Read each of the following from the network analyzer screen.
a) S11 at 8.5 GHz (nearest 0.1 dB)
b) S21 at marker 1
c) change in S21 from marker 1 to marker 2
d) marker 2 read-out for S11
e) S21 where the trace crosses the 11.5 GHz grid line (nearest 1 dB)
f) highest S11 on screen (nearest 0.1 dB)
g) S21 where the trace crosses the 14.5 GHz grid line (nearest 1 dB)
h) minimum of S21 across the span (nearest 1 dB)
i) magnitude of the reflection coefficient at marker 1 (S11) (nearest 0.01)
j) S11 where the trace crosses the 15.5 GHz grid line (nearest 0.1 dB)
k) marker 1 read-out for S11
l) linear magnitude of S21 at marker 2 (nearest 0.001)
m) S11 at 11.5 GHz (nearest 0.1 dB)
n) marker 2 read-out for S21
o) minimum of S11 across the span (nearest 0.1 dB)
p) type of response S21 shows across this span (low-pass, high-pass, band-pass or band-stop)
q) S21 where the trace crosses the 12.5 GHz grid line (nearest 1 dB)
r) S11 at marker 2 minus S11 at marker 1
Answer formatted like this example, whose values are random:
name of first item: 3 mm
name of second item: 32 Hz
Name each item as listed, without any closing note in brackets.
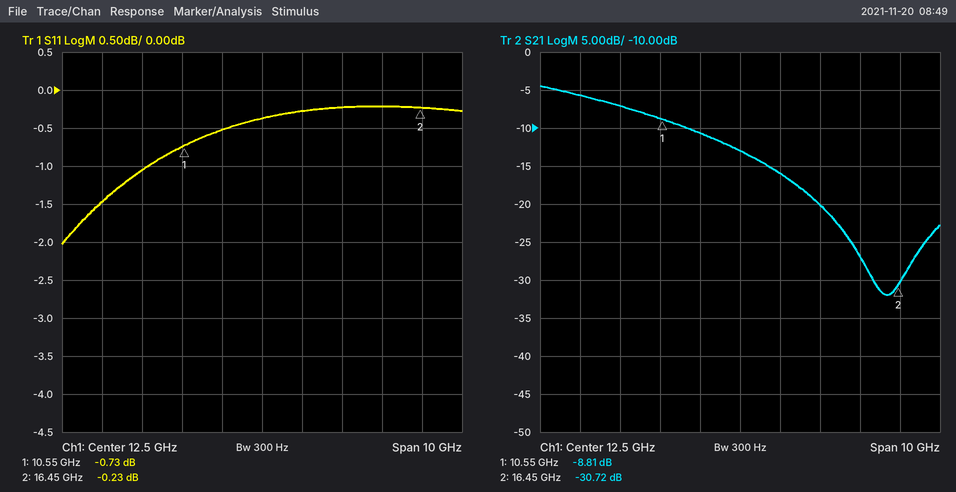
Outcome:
S11 at 8.5 GHz: -1.5 dB
S21 at marker 1: -8.81 dB
change in S21 from marker 1 to marker 2: -21.91 dB
marker 2 read-out for S11: -0.23 dB
S21 where the trace crosses the 11.5 GHz grid line: -11 dB
highest S11 on screen: -0.2 dB
S21 where the trace crosses the 14.5 GHz grid line: -20 dB
minimum of S21 across the span: -32 dB
magnitude of the reflection coefficient at marker 1 (S11): 0.92
S11 where the trace crosses the 15.5 GHz grid line: -0.2 dB
marker 1 read-out for S11: -0.73 dB
linear magnitude of S21 at marker 2: 0.029
S11 at 11.5 GHz: -0.5 dB
marker 2 read-out for S21: -30.72 dB
minimum of S11 across the span: -2.0 dB
type of response S21 shows across this span: low-pass
S21 where the trace crosses the 12.5 GHz grid line: -13 dB
S11 at marker 2 minus S11 at marker 1: 0.50 dB
